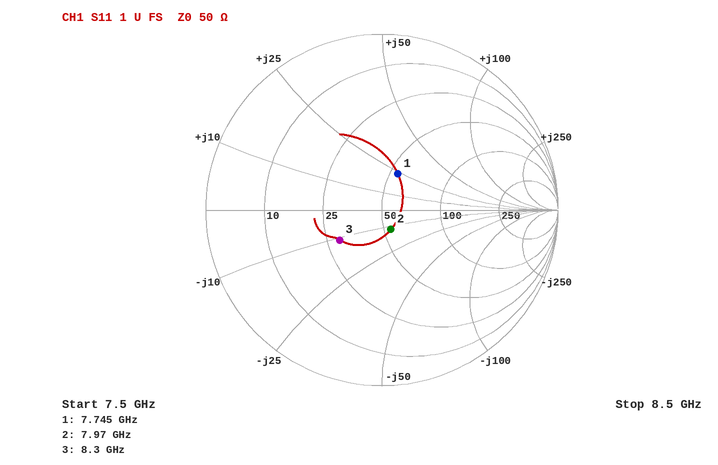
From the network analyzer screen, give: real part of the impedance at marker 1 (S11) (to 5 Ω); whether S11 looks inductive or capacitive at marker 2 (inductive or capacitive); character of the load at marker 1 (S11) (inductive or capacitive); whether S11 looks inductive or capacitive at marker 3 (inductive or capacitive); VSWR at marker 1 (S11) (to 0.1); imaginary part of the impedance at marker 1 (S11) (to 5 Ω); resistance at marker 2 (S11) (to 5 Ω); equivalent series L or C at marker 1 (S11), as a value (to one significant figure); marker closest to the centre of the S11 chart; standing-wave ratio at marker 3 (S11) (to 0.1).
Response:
55 Ω
capacitive
inductive
capacitive
1.6
+25 Ω
55 Ω
500 pH
marker 2
1.8
